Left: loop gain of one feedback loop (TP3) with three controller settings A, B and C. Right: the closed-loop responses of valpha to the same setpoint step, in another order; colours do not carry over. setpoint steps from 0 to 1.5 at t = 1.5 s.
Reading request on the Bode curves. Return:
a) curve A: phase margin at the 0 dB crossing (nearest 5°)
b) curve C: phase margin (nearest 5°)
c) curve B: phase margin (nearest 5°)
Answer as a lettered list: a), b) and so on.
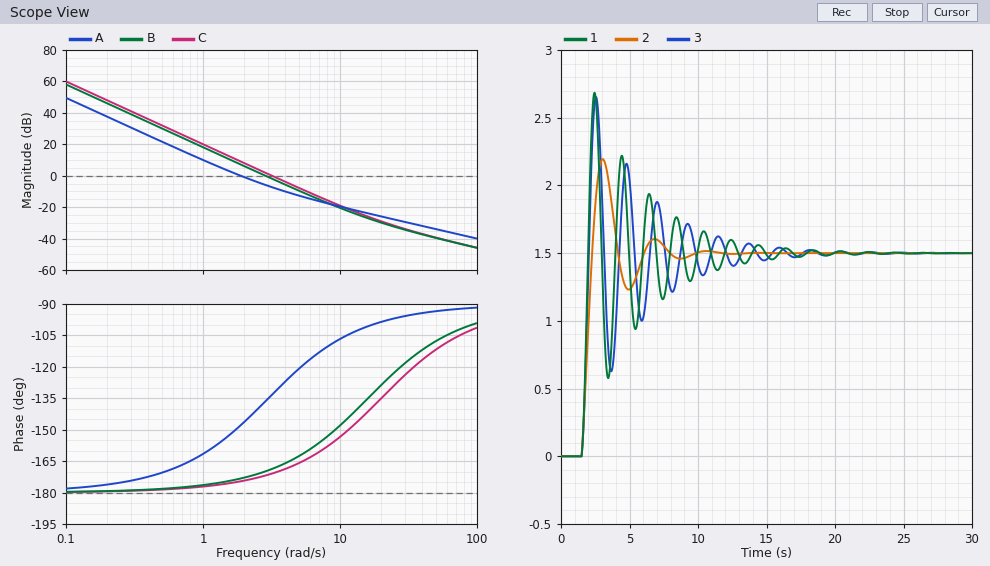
a) 30°
b) 10°
c) 10°
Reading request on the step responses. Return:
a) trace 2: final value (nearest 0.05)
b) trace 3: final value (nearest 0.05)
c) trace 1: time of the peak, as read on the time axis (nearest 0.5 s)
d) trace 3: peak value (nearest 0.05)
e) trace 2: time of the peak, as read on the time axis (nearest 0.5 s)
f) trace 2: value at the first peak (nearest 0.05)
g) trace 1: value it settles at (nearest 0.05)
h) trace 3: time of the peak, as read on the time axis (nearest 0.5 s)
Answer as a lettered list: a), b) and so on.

a) 1.50
b) 1.50
c) 2.5 s
d) 2.65
e) 3.0 s
f) 2.20
g) 1.50
h) 2.5 s
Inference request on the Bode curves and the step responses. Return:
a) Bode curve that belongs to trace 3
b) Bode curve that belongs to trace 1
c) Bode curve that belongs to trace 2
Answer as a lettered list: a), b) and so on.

a) B
b) C
c) A
